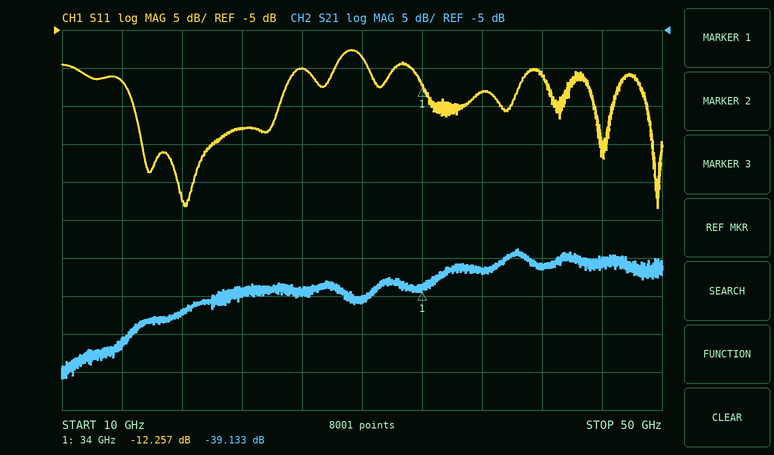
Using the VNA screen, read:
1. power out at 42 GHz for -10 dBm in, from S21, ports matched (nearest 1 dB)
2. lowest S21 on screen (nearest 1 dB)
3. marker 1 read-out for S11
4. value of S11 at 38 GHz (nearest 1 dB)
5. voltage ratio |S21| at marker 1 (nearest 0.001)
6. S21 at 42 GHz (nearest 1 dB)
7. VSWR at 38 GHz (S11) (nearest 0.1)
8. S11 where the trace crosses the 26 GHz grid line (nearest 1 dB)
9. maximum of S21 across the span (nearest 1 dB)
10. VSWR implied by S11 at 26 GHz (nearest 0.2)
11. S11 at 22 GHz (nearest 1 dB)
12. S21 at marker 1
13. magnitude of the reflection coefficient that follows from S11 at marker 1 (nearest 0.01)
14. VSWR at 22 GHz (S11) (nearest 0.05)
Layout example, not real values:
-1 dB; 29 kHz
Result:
-46 dBm; -51 dB; -12.257 dB; -13 dB; 0.011; -36 dB; 1.6; -10 dB; -34 dB; 2.0; -18 dB; -39.133 dB; 0.24; 1.30
